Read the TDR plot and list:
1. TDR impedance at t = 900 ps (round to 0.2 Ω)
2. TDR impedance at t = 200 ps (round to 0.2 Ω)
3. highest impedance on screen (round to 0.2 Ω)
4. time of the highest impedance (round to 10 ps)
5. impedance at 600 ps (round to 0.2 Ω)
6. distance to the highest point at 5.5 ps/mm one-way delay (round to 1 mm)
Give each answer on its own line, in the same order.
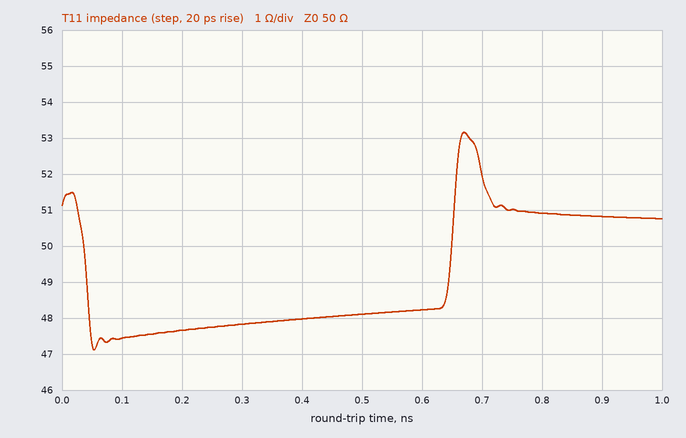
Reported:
50.8 Ω
47.6 Ω
53.2 Ω
670 ps
48.2 Ω
61 mm
